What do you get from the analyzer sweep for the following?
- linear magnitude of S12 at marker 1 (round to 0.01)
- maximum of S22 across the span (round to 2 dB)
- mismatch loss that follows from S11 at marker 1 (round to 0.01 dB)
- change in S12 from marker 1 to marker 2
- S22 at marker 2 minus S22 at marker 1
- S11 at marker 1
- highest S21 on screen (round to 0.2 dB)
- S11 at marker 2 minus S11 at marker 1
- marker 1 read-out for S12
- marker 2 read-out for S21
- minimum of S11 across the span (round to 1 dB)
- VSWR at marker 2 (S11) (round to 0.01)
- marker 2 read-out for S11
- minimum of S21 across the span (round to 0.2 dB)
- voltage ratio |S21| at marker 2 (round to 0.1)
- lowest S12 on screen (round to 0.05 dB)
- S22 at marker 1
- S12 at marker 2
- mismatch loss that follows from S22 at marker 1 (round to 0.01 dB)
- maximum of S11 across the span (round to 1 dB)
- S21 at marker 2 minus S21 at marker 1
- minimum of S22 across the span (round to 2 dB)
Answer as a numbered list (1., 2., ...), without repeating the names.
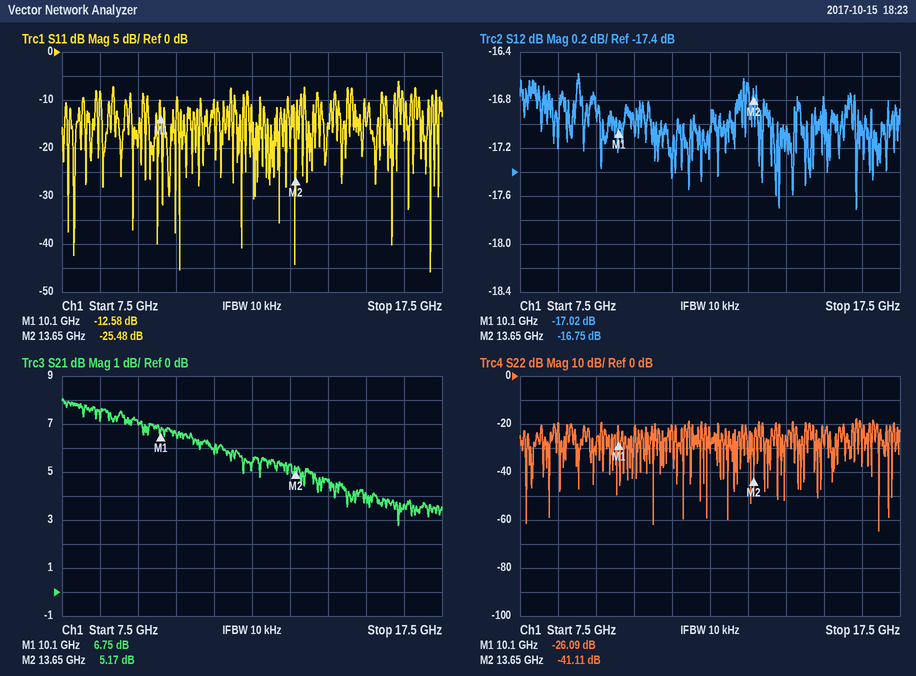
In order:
1. 0.14
2. -18 dB
3. 0.25 dB
4. 0.27 dB
5. -15.02 dB
6. -12.58 dB
7. 8.0 dB
8. -12.90 dB
9. -17.02 dB
10. 5.17 dB
11. -46 dB
12. 1.11
13. -25.48 dB
14. 2.8 dB
15. 1.8
16. -17.70 dB
17. -26.09 dB
18. -16.75 dB
19. 0.01 dB
20. -6 dB
21. -1.58 dB
22. -64 dB
